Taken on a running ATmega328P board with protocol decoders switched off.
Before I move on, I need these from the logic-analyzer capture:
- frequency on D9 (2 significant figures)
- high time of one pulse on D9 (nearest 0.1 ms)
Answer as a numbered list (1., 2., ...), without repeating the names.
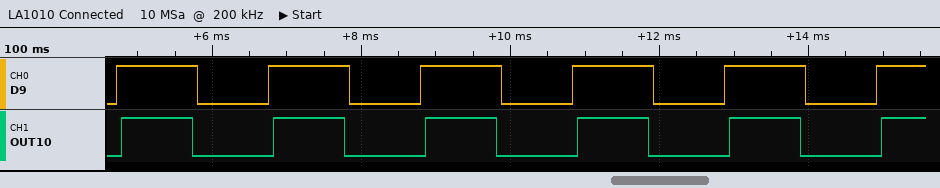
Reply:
1. 490 Hz
2. 1.1 ms
